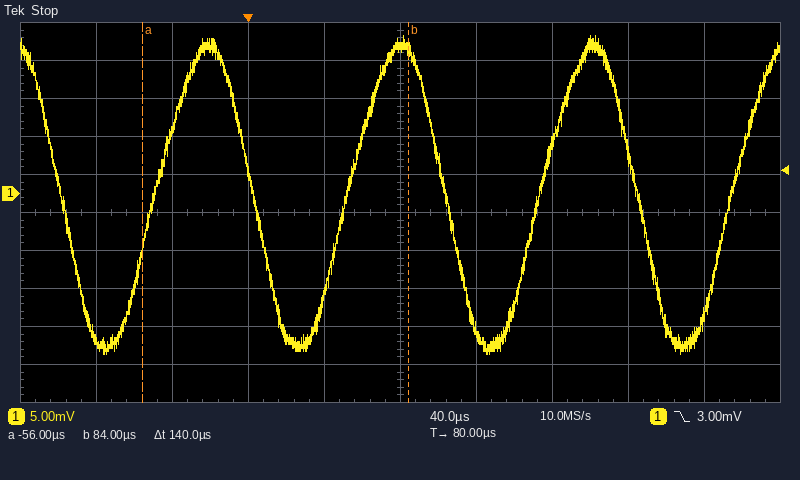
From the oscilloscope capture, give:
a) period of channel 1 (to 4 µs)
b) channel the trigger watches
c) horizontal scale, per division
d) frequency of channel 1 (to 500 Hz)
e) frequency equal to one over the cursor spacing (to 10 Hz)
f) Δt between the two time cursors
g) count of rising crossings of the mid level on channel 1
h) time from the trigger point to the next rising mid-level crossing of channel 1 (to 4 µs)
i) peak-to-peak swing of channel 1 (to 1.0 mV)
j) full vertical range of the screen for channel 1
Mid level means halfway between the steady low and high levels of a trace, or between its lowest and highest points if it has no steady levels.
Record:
100 µs
channel 1
40 µs
10.0 kHz
7.14 kHz
140 µs
4
52 µs
42.0 mV
50 mV
